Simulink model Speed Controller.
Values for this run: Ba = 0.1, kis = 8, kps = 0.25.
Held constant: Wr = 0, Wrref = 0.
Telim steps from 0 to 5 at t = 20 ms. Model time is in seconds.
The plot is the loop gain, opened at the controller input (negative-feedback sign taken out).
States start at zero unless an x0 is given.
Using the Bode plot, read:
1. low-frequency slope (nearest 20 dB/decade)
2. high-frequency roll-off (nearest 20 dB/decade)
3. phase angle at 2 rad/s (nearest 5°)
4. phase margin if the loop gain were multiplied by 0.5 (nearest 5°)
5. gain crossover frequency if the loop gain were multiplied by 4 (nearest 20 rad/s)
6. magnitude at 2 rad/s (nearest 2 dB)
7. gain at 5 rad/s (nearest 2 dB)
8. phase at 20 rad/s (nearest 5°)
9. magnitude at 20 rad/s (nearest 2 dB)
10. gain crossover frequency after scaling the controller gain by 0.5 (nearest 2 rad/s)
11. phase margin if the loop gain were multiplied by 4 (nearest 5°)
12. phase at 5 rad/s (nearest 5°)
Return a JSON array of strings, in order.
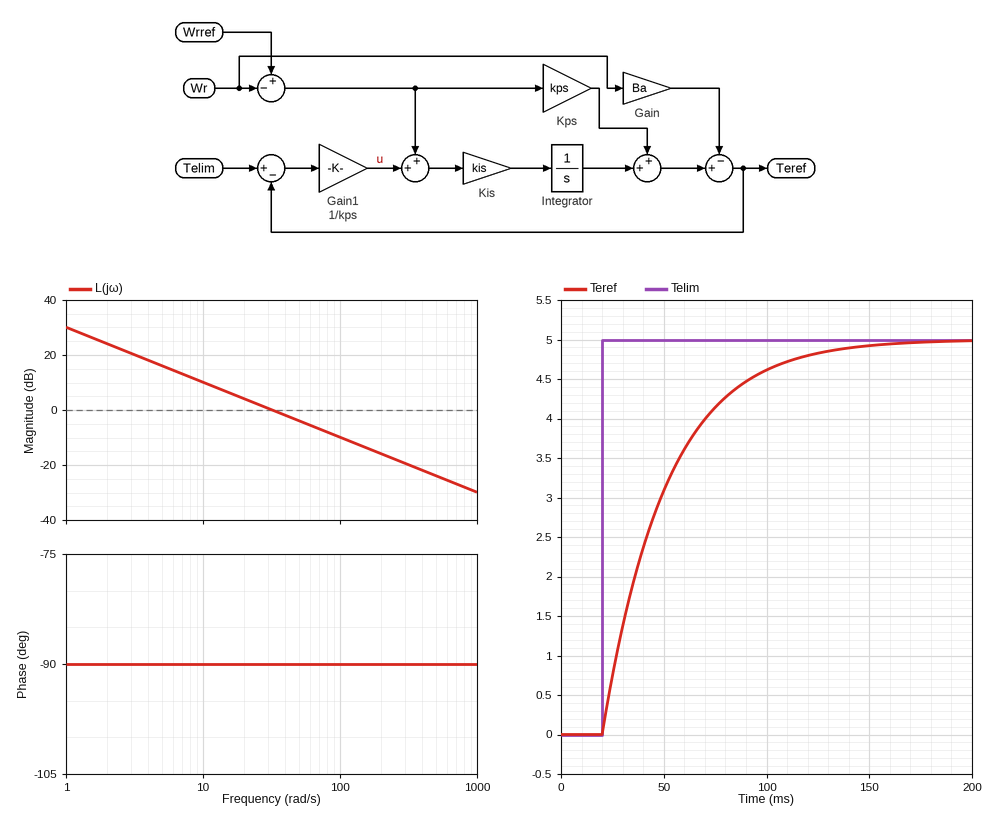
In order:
["-20 dB/decade", "-20 dB/decade", "-90°", "90°", "120 rad/s", "24 dB", "16 dB", "-90°", "4 dB", "16 rad/s", "90°", "-90°"]
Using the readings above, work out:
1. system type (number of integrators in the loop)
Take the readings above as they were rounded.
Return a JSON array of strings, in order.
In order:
["1"]
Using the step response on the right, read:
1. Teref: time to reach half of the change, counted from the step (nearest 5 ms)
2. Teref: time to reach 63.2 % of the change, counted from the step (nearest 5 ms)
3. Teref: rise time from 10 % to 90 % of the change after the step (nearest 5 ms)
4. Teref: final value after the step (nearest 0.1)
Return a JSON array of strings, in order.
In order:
["20 ms", "30 ms", "70 ms", "5.0"]
